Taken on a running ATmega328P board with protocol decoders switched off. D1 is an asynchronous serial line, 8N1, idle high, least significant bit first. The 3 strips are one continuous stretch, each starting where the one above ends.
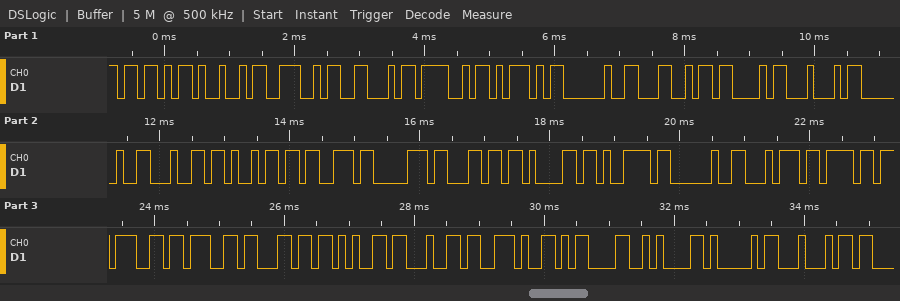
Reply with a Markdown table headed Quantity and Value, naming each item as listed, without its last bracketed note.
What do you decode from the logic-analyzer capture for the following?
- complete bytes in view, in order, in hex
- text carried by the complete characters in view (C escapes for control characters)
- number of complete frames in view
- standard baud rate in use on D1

| Quantity | Value |
|---|---|
| complete bytes in view, in order, in hex | 0x5B 0x49 0x4E 0x46 0x4F 0x5D 0x20 0x4C 0x43 0x44 0x20 0x64 0x69 0x73 0x70 0x6C 0x61 0x79 0x20 0x74 0x6F 0x67 0x67 0x6C 0x65 0x64 0x2E 0x0D 0x0A 0x41 0x44 |
| text carried by the complete characters in view | "[INFO] LCD display toggled.\r\nAD" |
| number of complete frames in view | 31 |
| standard baud rate in use on D1 | 9600 baud |
